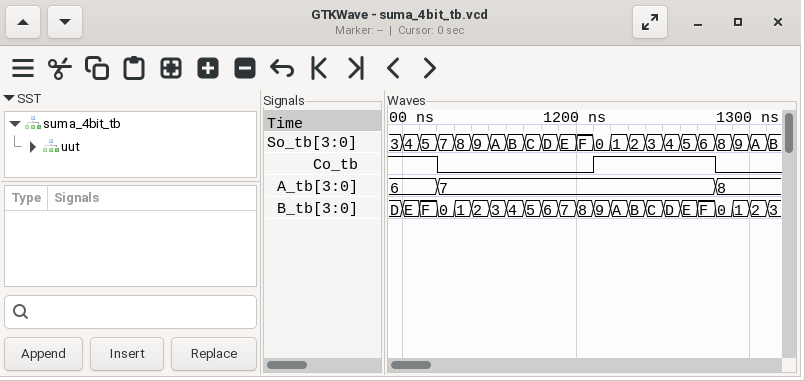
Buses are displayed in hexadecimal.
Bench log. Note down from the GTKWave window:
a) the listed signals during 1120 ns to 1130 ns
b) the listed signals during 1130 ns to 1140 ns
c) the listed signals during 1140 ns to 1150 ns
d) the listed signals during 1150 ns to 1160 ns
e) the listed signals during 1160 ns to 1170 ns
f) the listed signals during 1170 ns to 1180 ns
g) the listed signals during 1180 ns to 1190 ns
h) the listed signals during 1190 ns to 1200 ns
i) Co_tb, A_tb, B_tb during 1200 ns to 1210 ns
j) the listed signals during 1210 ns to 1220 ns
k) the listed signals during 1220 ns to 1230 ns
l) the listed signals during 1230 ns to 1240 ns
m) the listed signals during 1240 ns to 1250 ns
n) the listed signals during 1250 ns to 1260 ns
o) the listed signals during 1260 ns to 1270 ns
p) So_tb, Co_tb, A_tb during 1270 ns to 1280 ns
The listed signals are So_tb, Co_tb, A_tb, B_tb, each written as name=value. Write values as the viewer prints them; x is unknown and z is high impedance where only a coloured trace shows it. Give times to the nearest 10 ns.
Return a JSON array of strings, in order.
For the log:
["So_tb=7, Co_tb=0, A_tb=7, B_tb=0", "So_tb=8, Co_tb=0, A_tb=7, B_tb=1", "So_tb=9, Co_tb=0, A_tb=7, B_tb=2", "So_tb=A, Co_tb=0, A_tb=7, B_tb=3", "So_tb=B, Co_tb=0, A_tb=7, B_tb=4", "So_tb=C, Co_tb=0, A_tb=7, B_tb=5", "So_tb=D, Co_tb=0, A_tb=7, B_tb=6", "So_tb=E, Co_tb=0, A_tb=7, B_tb=7", "Co_tb=0, A_tb=7, B_tb=8", "So_tb=0, Co_tb=1, A_tb=7, B_tb=9", "So_tb=1, Co_tb=1, A_tb=7, B_tb=A", "So_tb=2, Co_tb=1, A_tb=7, B_tb=B", "So_tb=3, Co_tb=1, A_tb=7, B_tb=C", "So_tb=4, Co_tb=1, A_tb=7, B_tb=D", "So_tb=5, Co_tb=1, A_tb=7, B_tb=E", "So_tb=6, Co_tb=1, A_tb=7"]
